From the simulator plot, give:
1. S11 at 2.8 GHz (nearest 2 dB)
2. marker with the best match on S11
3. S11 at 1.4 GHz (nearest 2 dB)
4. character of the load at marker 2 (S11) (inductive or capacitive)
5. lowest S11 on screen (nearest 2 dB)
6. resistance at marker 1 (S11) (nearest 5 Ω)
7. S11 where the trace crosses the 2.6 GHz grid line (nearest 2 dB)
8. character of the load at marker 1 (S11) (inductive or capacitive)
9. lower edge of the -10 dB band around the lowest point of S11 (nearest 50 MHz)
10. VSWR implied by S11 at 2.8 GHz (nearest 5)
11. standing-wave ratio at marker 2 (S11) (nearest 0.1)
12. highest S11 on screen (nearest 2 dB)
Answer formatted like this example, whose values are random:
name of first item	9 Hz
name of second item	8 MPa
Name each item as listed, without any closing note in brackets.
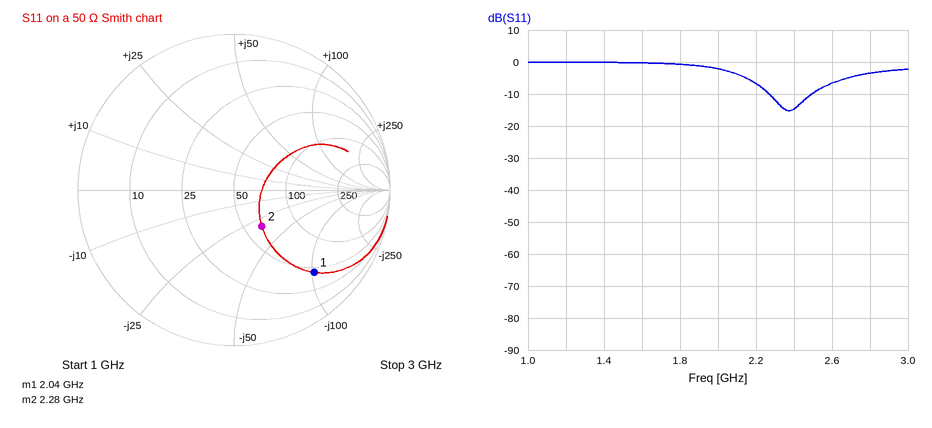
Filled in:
S11 at 2.8 GHz	-4 dB
marker with the best match on S11	marker 2
S11 at 1.4 GHz	0 dB
character of the load at marker 2 (S11)	capacitive
lowest S11 on screen	-16 dB
resistance at marker 1 (S11)	45 Ω
S11 where the trace crosses the 2.6 GHz grid line	-6 dB
character of the load at marker 1 (S11)	capacitive
lower edge of the -10 dB band around the lowest point of S11	2.25 GHz
VSWR implied by S11 at 2.8 GHz	5
standing-wave ratio at marker 2 (S11)	1.8
highest S11 on screen	0 dB
